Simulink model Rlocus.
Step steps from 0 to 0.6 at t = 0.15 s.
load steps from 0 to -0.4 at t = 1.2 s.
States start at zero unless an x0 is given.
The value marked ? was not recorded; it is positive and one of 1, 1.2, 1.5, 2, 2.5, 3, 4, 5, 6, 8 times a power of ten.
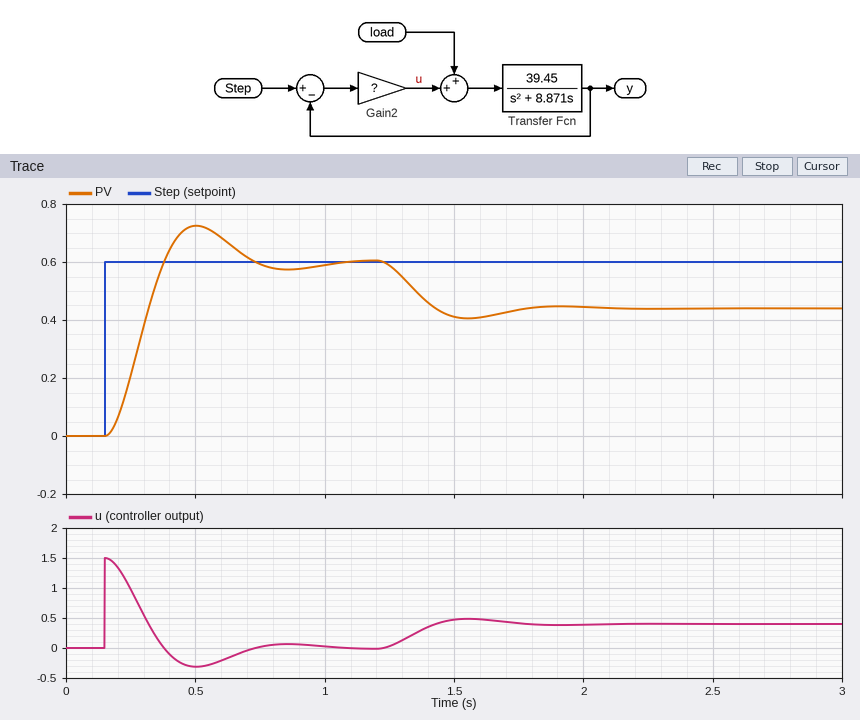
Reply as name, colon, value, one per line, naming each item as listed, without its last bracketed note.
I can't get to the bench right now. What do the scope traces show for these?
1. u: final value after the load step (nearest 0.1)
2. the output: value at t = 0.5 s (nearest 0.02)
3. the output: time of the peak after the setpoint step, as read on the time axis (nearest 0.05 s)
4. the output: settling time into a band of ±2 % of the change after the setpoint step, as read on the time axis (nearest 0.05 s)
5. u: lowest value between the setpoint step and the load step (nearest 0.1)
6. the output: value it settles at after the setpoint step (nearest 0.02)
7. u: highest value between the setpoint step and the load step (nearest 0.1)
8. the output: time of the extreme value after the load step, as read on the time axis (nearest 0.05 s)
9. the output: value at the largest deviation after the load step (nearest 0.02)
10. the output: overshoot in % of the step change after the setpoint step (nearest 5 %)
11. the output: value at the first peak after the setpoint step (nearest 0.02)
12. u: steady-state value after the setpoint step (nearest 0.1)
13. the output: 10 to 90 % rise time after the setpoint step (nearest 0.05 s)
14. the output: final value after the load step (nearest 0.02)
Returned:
u: final value after the load step: 0.4
the output: value at t = 0.5 s: 0.72
the output: time of the peak after the setpoint step, as read on the time axis: 0.50 s
the output: settling time into a band of ±2 % of the change after the setpoint step, as read on the time axis: 1.00 s
u: lowest value between the setpoint step and the load step: -0.3
the output: value it settles at after the setpoint step: 0.60
u: highest value between the setpoint step and the load step: 1.5
the output: time of the extreme value after the load step, as read on the time axis: 1.55 s
the output: value at the largest deviation after the load step: 0.40
the output: overshoot in % of the step change after the setpoint step: 20 %
the output: value at the first peak after the setpoint step: 0.72
u: steady-state value after the setpoint step: 0.0
the output: 10 to 90 % rise time after the setpoint step: 0.15 s
the output: final value after the load step: 0.44
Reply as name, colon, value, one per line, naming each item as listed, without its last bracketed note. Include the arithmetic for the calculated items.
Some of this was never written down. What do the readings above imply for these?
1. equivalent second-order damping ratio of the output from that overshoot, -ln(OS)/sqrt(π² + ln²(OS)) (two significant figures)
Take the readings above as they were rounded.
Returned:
equivalent second-order damping ratio of the output from that overshoot, -ln(OS)/sqrt(π² + ln²(OS)): ln(0.2) = -1.609; 1.609 / sqrt(9.870 + 2.590) = 0.46
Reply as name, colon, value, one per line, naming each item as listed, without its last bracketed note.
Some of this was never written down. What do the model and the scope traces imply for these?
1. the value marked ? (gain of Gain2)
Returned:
the value marked ?: 2.5
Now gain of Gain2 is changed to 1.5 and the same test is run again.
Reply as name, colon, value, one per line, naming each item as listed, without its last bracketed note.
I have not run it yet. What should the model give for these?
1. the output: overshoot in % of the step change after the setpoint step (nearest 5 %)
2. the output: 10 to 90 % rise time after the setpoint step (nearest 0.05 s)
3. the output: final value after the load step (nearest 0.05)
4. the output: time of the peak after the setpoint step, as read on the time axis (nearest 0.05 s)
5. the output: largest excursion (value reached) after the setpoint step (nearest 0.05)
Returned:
the output: overshoot in % of the step change after the setpoint step: 10 %
the output: 10 to 90 % rise time after the setpoint step: 0.25 s
the output: final value after the load step: 0.35
the output: time of the peak after the setpoint step, as read on the time axis: 0.65 s
the output: largest excursion (value reached) after the setpoint step: 0.65
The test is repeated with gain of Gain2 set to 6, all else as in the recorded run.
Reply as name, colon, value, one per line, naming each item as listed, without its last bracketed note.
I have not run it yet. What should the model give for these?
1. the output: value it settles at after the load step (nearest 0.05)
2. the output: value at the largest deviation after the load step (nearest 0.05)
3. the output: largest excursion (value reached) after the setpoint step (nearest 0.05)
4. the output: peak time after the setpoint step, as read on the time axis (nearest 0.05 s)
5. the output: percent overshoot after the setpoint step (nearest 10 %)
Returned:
the output: value it settles at after the load step: 0.55
the output: value at the largest deviation after the load step: 0.50
the output: largest excursion (value reached) after the setpoint step: 0.85
the output: peak time after the setpoint step, as read on the time axis: 0.35 s
the output: percent overshoot after the setpoint step: 40 %
